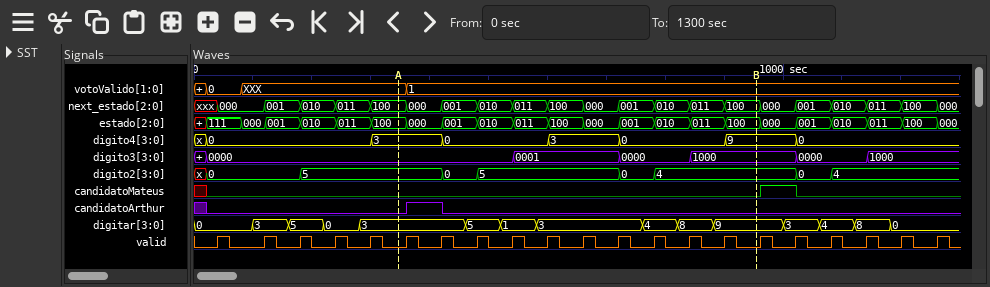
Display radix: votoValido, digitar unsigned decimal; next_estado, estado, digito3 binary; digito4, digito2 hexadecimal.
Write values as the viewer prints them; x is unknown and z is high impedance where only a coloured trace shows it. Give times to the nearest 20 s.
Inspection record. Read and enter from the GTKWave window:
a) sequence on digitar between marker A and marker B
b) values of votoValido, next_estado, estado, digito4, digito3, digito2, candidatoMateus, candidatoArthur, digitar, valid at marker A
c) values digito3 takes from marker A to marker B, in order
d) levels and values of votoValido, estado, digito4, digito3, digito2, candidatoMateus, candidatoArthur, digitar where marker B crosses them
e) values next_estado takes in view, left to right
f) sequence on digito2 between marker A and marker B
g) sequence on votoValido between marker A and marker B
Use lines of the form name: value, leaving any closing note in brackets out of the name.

sequence on digitar between marker A and marker B: 3, 5, 1, 3, 4, 8, 9
values of votoValido, next_estado, estado, digito4, digito3, digito2, candidatoMateus, candidatoArthur, digitar, valid at marker A: votoValido=XXX, next_estado=100, estado=100, digito4=3, digito3=0000, digito2=5, candidatoMateus=0, candidatoArthur=0, digitar=3, valid=0
values digito3 takes from marker A to marker B, in order: 0000, 0001, 0000, 1000
levels and values of votoValido, estado, digito4, digito3, digito2, candidatoMateus, candidatoArthur, digitar where marker B crosses them: votoValido=1, estado=100, digito4=9, digito3=1000, digito2=4, candidatoMateus=0, candidatoArthur=0, digitar=9
values next_estado takes in view, left to right: xxx, 000, 001, 010, 011, 100, 000, 001, 010, 011, 100, 000, 001, 010, 011, 100, 000, 001, 010, 011, 100, 000
sequence on digito2 between marker A and marker B: 5, 0, 5, 0, 4
sequence on votoValido between marker A and marker B: XXX, 1
